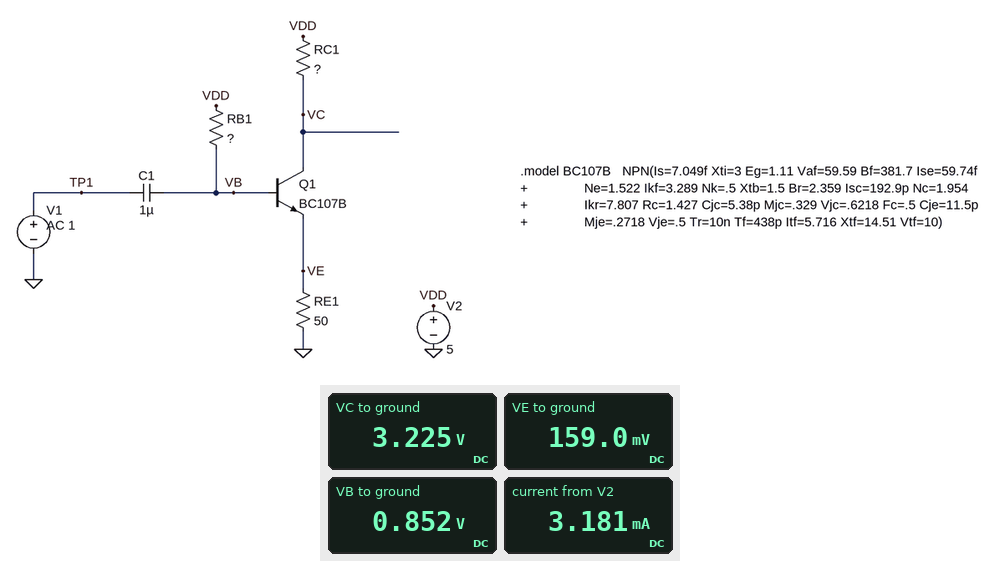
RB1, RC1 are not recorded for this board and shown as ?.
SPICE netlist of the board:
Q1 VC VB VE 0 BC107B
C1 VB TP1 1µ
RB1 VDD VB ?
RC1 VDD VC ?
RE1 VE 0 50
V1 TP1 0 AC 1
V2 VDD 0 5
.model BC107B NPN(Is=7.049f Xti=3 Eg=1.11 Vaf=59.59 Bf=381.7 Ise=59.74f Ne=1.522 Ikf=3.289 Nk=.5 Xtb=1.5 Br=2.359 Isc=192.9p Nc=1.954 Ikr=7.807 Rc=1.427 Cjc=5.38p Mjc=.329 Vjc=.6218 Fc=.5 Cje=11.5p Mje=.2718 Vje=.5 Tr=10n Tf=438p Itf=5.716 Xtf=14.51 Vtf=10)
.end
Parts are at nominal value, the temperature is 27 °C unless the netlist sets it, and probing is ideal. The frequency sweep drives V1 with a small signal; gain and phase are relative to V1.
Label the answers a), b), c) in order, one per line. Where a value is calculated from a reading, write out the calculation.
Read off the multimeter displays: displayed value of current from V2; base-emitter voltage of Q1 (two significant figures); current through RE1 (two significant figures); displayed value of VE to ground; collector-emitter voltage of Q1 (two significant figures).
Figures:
a) 3.181 mA
b) 852 mV - 159 mV = 690 mV
c) (159 mV) / 50 Ω = 3.2 mA
d) 159.0 mV
e) 3.225 V - 159 mV = 3.1 V
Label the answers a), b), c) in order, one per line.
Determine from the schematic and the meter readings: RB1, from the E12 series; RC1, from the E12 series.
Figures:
a) 390 kΩ
b) 560 Ω
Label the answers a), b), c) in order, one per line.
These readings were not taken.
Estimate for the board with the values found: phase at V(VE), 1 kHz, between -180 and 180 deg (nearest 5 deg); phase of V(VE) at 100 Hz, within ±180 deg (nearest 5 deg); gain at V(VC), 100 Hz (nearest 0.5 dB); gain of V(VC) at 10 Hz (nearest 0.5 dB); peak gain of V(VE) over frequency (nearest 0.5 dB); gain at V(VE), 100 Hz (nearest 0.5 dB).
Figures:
a) 0 deg
b) 5 deg
c) 19.5 dB
d) 17.0 dB
e) -1.5 dB
f) -1.5 dB
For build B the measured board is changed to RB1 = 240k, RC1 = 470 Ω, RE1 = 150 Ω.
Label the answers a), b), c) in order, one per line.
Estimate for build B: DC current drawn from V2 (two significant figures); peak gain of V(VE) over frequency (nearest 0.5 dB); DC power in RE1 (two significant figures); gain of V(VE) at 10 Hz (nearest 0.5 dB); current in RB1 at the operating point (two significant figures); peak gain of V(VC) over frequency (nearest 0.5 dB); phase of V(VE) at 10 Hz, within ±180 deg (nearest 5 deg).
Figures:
a) 4.6 mA
b) -0.5 dB
c) 3.1 mW
d) -1.0 dB
e) 15 µA
f) 9.5 dB
g) 20 deg
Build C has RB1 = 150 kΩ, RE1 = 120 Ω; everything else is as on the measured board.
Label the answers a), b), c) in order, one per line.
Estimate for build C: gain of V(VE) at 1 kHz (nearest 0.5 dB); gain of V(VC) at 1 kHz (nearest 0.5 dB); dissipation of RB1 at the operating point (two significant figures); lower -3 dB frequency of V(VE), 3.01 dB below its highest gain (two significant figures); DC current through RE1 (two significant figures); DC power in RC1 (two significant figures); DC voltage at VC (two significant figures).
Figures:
a) -0.5 dB
b) 13.0 dB
c) 80 µW
d) 13 Hz
e) 6.9 mA
f) 26 mW
g) 1.2 V
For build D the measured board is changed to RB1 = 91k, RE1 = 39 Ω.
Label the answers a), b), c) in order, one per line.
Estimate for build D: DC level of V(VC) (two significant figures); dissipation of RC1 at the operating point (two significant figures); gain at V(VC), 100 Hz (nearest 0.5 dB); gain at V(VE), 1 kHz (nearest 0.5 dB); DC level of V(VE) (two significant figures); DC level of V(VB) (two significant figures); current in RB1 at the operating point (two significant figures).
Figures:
a) 490 mV
b) 36 mW
c) 2.0 dB
d) -3.0 dB
e) 320 mV
f) 1.0 V
g) 44 µA
